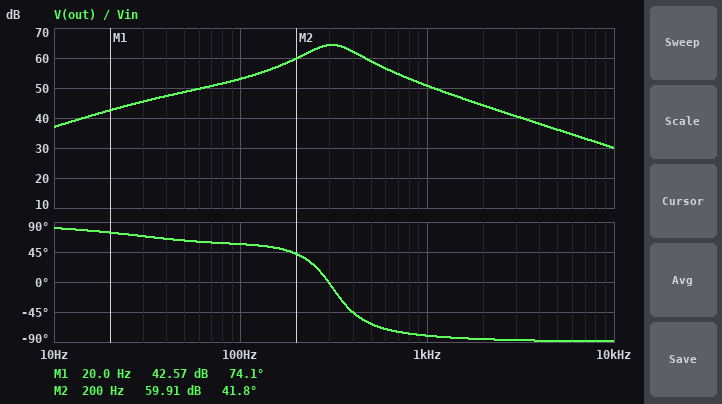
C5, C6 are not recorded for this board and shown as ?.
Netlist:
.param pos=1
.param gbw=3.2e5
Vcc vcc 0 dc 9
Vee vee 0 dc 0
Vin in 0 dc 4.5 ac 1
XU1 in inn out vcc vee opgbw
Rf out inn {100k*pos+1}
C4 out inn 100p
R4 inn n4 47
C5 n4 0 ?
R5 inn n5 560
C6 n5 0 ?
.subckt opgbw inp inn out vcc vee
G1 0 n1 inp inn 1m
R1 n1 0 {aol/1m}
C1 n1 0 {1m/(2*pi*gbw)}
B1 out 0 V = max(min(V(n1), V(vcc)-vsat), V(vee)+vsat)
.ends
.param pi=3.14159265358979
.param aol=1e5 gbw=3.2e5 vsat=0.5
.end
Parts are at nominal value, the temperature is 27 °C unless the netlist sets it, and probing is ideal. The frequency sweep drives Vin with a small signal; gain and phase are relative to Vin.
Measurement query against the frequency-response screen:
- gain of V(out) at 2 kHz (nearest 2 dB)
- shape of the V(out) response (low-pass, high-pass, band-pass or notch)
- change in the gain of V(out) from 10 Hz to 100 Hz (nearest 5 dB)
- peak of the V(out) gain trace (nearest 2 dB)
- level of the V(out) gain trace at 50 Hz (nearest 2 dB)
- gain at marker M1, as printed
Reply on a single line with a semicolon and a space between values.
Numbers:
44 dB; band-pass; 15 dB; 64 dB; 48 dB; 42.57 dB
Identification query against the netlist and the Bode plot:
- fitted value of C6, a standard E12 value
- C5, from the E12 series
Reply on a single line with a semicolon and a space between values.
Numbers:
6.8 µF; 4.7 µF
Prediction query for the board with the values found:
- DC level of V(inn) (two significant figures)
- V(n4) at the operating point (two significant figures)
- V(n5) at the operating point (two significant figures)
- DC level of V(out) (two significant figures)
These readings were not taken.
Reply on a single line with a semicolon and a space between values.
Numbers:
4.5 V; 4.5 V; 4.5 V; 4.5 V
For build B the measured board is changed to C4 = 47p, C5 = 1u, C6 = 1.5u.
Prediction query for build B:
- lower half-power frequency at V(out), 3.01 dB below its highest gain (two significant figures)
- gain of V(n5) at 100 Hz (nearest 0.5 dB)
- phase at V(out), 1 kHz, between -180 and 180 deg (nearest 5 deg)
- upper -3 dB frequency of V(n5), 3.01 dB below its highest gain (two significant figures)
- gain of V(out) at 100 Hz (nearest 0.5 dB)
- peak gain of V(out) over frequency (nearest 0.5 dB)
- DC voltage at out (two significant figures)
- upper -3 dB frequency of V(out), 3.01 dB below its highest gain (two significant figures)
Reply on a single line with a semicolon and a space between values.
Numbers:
460 Hz; -0.5 dB; -70 deg; 290 Hz; 43.5 dB; 59.5 dB; 4.5 V; 840 Hz
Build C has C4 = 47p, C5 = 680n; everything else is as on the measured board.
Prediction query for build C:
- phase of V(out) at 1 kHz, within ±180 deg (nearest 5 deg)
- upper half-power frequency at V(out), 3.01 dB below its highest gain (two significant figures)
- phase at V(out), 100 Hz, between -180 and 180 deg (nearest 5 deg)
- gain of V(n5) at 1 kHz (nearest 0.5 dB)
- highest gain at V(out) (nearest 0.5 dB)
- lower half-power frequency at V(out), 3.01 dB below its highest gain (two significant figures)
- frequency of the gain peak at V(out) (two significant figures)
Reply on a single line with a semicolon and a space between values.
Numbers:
-50 deg; 1.1 kHz; 30 deg; -26.5 dB; 56.5 dB; 550 Hz; 800 Hz
